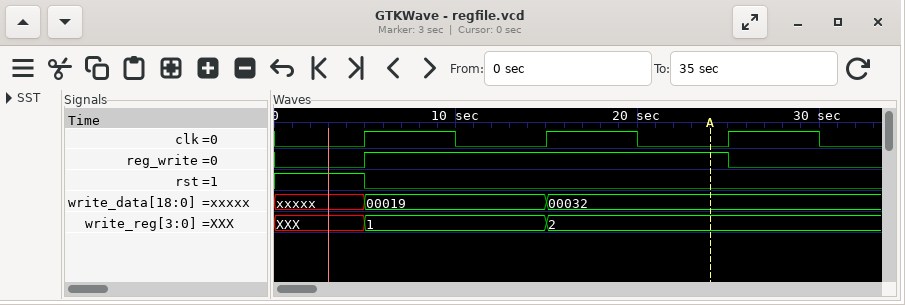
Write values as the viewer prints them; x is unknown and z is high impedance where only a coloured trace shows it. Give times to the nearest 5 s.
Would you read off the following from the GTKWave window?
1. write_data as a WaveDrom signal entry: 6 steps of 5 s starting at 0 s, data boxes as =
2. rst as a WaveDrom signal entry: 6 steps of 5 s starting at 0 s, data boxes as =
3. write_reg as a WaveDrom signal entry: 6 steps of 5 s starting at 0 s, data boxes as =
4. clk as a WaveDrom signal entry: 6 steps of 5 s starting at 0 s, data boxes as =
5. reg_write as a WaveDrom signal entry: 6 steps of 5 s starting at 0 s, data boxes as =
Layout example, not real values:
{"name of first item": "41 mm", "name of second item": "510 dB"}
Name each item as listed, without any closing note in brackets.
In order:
{"write_data as a WaveDrom signal entry: 6 steps of 5 s starting at 0 s, data boxes as =": "{name: 'write_data', wave: 'x=.=..', data: '00019 00032'}", "rst as a WaveDrom signal entry: 6 steps of 5 s starting at 0 s, data boxes as =": "{name: 'rst', wave: '10....'}", "write_reg as a WaveDrom signal entry: 6 steps of 5 s starting at 0 s, data boxes as =": "{name: 'write_reg', wave: 'x=.=..', data: '1 2'}", "clk as a WaveDrom signal entry: 6 steps of 5 s starting at 0 s, data boxes as =": "{name: 'clk', wave: '010101'}", "reg_write as a WaveDrom signal entry: 6 steps of 5 s starting at 0 s, data boxes as =": "{name: 'reg_write', wave: '01...0'}"}
